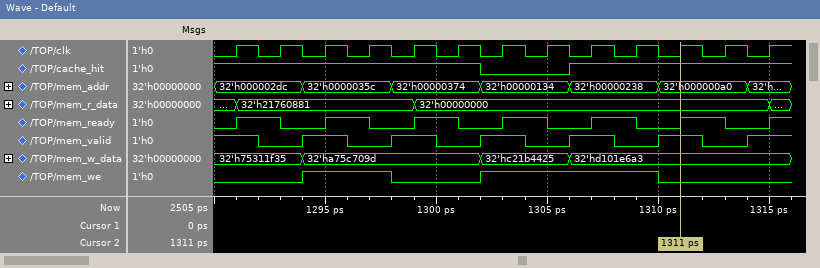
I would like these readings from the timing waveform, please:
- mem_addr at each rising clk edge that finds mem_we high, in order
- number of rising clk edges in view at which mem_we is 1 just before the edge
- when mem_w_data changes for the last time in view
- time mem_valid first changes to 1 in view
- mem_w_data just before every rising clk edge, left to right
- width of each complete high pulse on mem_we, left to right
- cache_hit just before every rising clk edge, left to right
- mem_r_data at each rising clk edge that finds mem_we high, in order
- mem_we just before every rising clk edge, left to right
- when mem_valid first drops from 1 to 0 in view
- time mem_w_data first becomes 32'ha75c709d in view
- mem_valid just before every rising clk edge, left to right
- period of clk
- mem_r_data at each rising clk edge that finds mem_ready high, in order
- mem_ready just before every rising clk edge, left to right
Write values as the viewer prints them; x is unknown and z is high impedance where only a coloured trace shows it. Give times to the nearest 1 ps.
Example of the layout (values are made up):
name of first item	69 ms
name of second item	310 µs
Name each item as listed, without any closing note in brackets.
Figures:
mem_addr at each rising clk edge that finds mem_we high, in order	32'h0000035c, 32'h0000035c, 32'h00000134, 32'h00000134, 32'h00000238, 32'h00000238
number of rising clk edges in view at which mem_we is 1 just before the edge	6
when mem_w_data changes for the last time in view	1306 ps
time mem_valid first changes to 1 in view	1294 ps
mem_w_data just before every rising clk edge, left to right	32'h75311f35, 32'h75311f35, 32'ha75c709d, 32'ha75c709d, 32'ha75c709d, 32'ha75c709d, 32'hc21b4425, 32'hc21b4425, 32'hd101e6a3, 32'hd101e6a3, 32'hd101e6a3, 32'hd101e6a3, 32'hd101e6a3
width of each complete high pulse on mem_we, left to right	4 ps, 8 ps
cache_hit just before every rising clk edge, left to right	1 1 1 1 1 1 0 0 1 1 1 1 1
mem_r_data at each rising clk edge that finds mem_we high, in order	32'h21760881, 32'h21760881, 32'h00000000, 32'h00000000, 32'h00000000, 32'h00000000
mem_we just before every rising clk edge, left to right	0 0 1 1 0 0 1 1 1 1 0 0 0
when mem_valid first drops from 1 to 0 in view	1292 ps
time mem_w_data first becomes 32'ha75c709d in view	1294 ps
mem_valid just before every rising clk edge, left to right	1 0 1 0 1 0 1 0 1 0 1 0 1
period of clk	2 ps
mem_r_data at each rising clk edge that finds mem_ready high, in order	32'h21760881, 32'h21760881, 32'h00000000, 32'h00000000, 32'h00000000, 32'h00000000
mem_ready just before every rising clk edge, left to right	0 1 0 1 0 1 0 1 0 1 0 1 0
